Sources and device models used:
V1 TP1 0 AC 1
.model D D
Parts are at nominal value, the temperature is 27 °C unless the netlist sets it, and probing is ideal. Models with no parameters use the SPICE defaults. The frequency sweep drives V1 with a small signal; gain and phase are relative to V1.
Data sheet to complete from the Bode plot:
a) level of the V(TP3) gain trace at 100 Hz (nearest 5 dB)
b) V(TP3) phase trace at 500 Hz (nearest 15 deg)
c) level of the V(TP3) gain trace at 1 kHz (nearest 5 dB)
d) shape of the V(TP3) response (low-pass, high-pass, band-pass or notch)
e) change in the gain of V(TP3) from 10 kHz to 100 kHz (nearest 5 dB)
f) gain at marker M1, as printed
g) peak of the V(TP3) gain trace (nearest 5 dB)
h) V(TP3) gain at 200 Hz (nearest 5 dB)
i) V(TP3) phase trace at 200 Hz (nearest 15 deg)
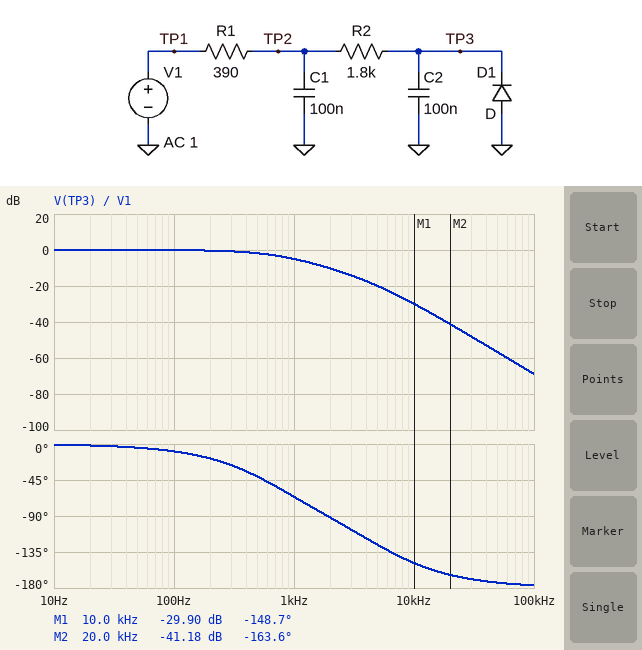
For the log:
0 dB
-45 deg
-5 dB
low-pass
-40 dB
-29.90 dB
0 dB
0 dB
-15 deg
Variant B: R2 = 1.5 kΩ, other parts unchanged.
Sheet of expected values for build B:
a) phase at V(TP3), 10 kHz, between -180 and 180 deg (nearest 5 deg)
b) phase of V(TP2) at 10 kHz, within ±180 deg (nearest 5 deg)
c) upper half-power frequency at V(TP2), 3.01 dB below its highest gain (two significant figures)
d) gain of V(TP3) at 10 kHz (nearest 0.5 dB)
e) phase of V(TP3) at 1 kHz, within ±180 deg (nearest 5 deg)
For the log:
-145 deg
-65 deg
2.5 kHz
-28.5 dB
-60 deg
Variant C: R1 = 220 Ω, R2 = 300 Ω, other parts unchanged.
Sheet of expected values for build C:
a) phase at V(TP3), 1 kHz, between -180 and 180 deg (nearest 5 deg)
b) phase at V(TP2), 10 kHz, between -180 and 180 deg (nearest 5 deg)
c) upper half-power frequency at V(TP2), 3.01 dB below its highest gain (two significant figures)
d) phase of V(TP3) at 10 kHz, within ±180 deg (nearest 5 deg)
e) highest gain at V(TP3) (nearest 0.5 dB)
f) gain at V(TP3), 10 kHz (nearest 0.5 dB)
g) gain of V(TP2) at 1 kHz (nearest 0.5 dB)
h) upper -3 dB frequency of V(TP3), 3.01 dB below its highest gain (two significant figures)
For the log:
-25 deg
-45 deg
3.2 kHz
-110 deg
0 dB
-14.0 dB
-0.5 dB
2.4 kHz
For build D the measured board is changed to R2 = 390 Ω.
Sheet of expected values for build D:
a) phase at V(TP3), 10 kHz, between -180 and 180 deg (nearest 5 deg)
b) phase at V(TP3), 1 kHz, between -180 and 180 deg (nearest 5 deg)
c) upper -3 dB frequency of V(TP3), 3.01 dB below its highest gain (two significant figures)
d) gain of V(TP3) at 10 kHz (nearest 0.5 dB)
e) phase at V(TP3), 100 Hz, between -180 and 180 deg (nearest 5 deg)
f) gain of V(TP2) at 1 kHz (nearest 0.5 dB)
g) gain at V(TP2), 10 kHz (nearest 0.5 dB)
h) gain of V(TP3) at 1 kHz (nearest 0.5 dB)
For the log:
-125 deg
-40 deg
1.5 kHz
-19.0 dB
-5 deg
-1.5 dB
-10.5 dB
-1.5 dB
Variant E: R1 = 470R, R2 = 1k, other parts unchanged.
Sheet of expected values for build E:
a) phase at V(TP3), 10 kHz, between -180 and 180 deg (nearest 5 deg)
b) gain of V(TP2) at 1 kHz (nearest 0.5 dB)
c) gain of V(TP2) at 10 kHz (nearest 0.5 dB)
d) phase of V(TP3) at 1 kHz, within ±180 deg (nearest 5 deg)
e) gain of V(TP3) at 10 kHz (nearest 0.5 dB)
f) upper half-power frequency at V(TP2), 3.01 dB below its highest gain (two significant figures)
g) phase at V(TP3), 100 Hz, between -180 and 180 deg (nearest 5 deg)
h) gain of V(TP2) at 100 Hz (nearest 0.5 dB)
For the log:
-145 deg
-2.0 dB
-10.5 dB
-55 deg
-26.5 dB
1.6 kHz
-5 deg
0 dB
